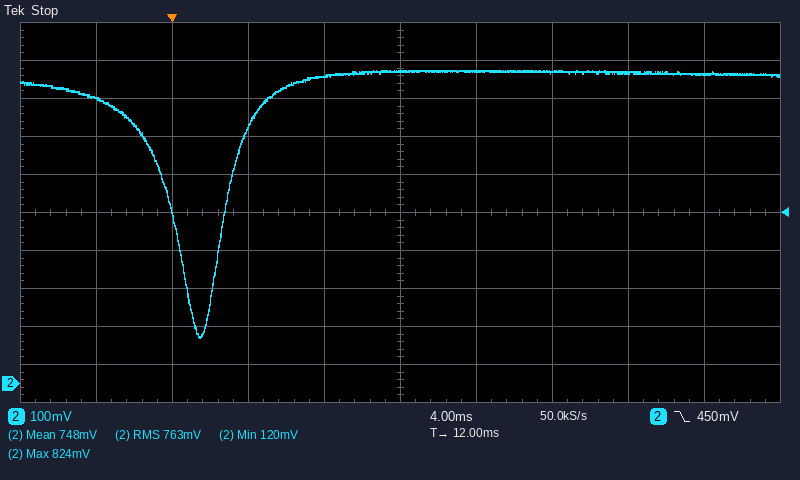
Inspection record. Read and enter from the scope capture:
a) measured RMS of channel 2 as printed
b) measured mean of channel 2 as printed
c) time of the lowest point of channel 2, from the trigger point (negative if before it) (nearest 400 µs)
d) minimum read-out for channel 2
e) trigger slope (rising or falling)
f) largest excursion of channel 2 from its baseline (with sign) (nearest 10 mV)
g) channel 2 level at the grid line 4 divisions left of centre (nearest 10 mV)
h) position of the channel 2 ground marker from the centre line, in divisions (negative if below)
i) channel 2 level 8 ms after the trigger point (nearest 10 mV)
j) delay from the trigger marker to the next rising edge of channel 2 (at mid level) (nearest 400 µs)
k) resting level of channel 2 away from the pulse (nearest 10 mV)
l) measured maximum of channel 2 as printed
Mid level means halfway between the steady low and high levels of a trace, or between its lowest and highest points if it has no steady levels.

763 mV
748 mV
+1.6 ms
120 mV
falling
-700 mV
750 mV
-4.5 div
810 mV
2.8 ms
820 mV
824 mV
